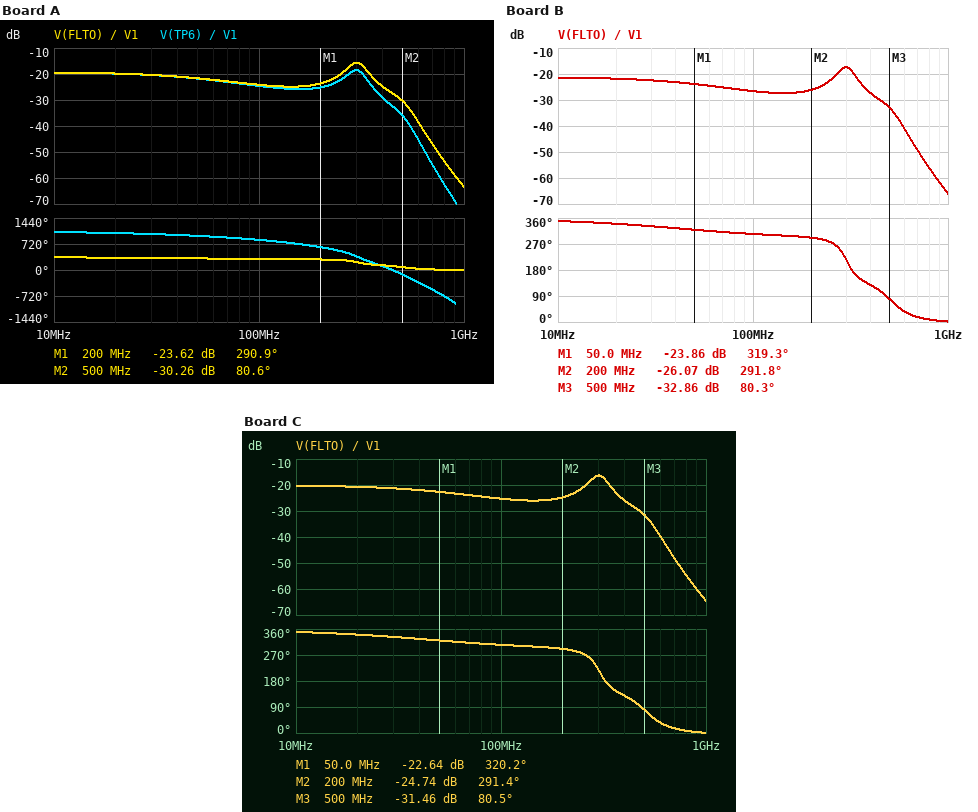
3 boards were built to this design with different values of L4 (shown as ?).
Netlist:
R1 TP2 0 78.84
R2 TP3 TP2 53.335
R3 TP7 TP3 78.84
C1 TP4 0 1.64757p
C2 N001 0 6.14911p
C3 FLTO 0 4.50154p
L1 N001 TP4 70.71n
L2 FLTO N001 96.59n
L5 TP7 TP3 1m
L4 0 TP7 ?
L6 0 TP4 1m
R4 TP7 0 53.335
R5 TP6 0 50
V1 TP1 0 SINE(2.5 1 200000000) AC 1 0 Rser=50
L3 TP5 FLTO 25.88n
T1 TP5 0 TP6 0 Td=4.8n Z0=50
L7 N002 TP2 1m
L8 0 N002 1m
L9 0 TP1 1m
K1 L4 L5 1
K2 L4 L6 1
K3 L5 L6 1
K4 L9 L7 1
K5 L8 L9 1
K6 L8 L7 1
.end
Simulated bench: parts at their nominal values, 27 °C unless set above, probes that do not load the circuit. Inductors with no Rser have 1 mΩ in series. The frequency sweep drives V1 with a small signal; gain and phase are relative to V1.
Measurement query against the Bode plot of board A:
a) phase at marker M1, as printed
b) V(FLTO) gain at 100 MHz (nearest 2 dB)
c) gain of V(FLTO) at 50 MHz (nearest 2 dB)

290.9 deg
-24 dB
-22 dB
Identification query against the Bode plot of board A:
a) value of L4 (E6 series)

1.5 mH
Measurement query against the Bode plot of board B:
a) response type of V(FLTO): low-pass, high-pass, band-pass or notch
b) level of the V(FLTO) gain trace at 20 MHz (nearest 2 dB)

low-pass
-22 dB
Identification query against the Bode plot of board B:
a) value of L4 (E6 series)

3.3 mH
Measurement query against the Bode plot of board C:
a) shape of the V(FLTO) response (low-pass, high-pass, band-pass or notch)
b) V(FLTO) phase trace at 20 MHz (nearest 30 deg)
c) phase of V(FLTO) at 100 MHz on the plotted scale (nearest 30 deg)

low-pass
330 deg
300 deg
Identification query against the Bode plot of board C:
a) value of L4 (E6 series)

2.2 mH
